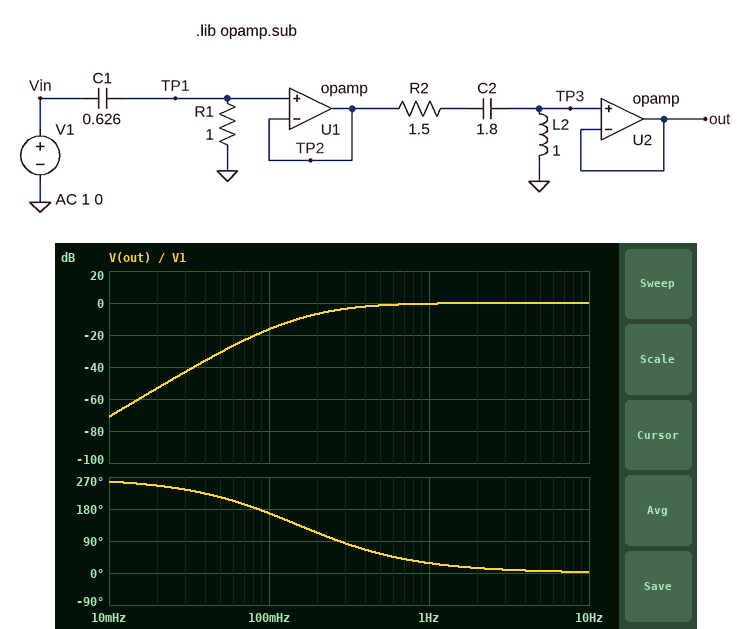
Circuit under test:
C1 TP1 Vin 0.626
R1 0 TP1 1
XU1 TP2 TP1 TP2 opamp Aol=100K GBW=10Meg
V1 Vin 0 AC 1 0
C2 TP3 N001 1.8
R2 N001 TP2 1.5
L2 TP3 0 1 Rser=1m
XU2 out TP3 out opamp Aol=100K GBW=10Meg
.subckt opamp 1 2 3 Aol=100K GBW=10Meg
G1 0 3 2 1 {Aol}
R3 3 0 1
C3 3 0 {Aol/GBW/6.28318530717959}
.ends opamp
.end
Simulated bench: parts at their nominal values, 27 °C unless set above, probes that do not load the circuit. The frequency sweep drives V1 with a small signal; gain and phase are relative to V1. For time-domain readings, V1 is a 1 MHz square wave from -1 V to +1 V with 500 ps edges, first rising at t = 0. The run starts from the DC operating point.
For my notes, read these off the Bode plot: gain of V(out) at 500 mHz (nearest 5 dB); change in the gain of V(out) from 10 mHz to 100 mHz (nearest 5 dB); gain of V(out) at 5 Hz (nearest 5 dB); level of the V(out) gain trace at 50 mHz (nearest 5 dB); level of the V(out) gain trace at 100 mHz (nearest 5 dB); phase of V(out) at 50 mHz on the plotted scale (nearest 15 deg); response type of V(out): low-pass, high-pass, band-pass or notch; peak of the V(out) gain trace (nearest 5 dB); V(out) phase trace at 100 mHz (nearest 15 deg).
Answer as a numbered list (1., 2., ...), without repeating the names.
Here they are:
1. 0 dB
2. 55 dB
3. 0 dB
4. -30 dB
5. -15 dB
6. 210 deg
7. high-pass
8. 0 dB
9. 165 deg
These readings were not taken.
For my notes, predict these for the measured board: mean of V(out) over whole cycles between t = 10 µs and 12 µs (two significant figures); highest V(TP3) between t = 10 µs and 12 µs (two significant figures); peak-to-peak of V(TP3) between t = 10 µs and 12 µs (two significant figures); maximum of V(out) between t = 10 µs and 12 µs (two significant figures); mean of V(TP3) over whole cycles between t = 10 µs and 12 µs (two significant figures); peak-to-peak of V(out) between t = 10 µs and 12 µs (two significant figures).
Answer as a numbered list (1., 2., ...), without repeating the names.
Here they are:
1. 1.0 V
2. 2.0 V
3. 2.0 V
4. 2.0 V
5. 1.0 V
6. 2.0 V
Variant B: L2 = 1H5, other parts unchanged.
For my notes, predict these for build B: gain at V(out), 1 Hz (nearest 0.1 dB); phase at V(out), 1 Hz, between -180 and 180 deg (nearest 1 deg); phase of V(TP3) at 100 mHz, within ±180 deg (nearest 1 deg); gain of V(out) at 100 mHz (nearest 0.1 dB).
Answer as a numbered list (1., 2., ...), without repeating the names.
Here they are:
1. -0.3 dB
2. 23 deg
3. 156 deg
4. -12.8 dB
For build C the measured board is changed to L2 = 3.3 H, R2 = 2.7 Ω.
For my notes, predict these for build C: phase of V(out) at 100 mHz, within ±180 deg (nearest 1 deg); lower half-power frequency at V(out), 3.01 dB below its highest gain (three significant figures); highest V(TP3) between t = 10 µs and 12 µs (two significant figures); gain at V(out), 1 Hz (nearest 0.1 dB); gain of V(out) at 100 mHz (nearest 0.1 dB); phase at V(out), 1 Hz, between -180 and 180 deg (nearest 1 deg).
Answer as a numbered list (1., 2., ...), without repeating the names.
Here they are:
1. 135 deg
2. 283 mHz
3. 2.0 V
4. -0.3 dB
5. -11.8 dB
6. 22 deg
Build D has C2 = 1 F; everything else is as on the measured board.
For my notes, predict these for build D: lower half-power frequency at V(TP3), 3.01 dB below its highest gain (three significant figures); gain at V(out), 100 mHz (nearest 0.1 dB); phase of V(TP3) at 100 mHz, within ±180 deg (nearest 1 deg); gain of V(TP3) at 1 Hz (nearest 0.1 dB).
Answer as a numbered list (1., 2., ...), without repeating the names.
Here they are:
1. 297 mHz
2. -17.8 dB
3. -169 deg
4. -0.3 dB
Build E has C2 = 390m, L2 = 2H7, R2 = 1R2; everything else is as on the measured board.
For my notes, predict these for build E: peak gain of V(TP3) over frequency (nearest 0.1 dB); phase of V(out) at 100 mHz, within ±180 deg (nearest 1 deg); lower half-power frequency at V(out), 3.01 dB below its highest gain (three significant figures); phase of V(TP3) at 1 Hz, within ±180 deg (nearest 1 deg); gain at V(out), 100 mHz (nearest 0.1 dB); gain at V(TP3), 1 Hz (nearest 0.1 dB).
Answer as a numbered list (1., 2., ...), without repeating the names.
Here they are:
1. 1.9 dB
2. -138 deg
3. 140 mHz
4. 18 deg
5. -12.7 dB
6. -0.1 dB
